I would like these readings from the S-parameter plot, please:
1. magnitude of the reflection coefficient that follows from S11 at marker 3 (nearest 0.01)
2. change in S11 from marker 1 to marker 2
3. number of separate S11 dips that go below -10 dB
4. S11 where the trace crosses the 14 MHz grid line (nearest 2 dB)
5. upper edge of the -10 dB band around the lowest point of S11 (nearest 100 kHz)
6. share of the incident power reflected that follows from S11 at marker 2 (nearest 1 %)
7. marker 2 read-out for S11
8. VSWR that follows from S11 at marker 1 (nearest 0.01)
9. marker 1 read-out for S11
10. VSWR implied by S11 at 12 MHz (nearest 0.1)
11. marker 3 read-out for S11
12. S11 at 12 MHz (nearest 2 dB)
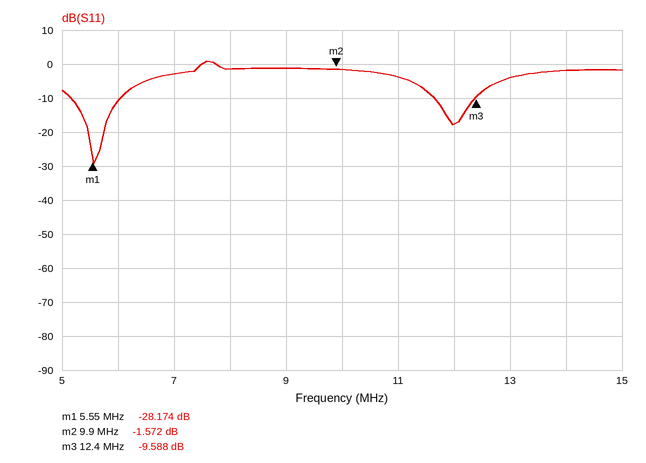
0.33
26.602 dB
2
-2 dB
6.0 MHz
70 %
-1.572 dB
1.08
-28.174 dB
1.3
-9.588 dB
-18 dB
